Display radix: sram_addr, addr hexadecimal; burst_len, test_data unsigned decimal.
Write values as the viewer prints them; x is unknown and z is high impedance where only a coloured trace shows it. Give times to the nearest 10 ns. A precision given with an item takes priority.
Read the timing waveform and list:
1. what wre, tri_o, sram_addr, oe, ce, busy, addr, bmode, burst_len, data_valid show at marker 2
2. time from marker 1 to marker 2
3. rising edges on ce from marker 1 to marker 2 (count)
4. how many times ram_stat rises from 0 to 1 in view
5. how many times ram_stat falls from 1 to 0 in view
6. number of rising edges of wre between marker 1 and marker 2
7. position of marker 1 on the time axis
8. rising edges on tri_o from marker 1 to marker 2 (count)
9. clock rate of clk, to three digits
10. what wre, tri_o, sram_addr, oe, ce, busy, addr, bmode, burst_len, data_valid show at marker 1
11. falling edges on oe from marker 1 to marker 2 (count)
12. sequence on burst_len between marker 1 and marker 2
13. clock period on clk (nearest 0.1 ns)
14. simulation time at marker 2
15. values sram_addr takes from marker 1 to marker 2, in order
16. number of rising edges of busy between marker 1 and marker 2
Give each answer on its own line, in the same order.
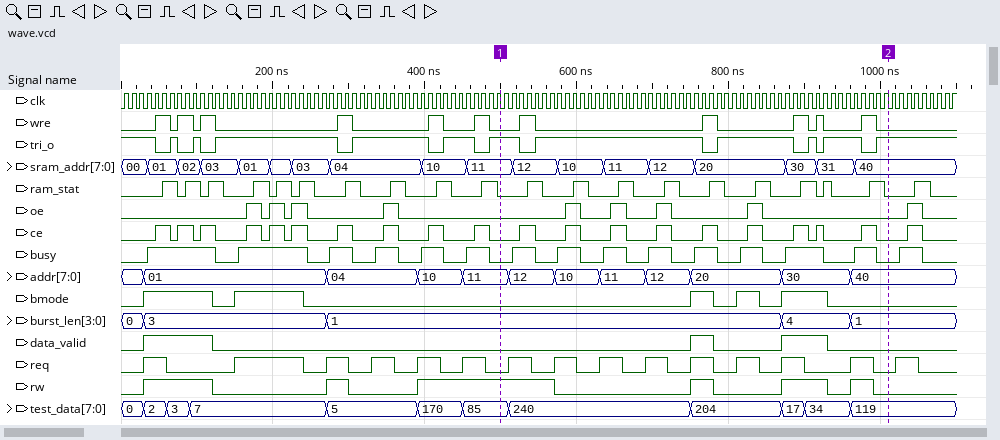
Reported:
wre=0, tri_o=1, sram_addr=40, oe=0, ce=0, busy=0, addr=40, bmode=0, burst_len=1, data_valid=0
510 ns
9
20
20
5
500 ns
5
100 MHz
wre=0, tri_o=1, sram_addr=11, oe=0, ce=0, busy=0, addr=11, bmode=0, burst_len=1, data_valid=0
4
1, 4, 1
10 ns
1010 ns
11, 12, 10, 11, 12, 20, 30, 31, 40
8
